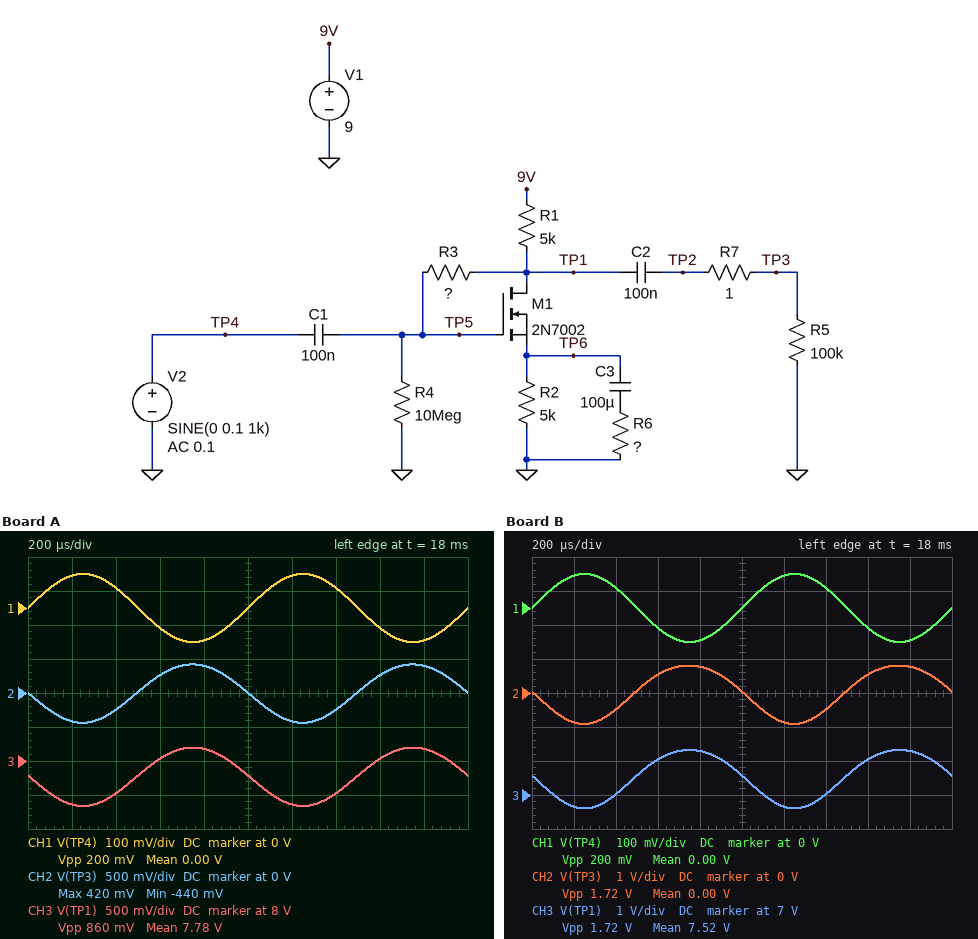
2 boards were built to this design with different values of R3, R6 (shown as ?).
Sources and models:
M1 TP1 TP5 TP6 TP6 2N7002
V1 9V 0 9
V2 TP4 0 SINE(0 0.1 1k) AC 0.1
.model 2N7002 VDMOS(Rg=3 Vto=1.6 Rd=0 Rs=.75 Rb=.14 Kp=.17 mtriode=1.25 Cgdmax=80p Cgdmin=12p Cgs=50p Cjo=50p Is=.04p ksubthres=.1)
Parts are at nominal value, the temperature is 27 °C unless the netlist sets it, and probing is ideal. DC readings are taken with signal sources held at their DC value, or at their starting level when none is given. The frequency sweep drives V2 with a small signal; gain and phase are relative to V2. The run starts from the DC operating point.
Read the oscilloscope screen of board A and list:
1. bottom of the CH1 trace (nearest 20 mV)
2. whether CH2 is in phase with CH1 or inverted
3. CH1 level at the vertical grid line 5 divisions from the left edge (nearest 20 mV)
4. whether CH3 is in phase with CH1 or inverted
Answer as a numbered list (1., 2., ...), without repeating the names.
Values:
1. -100 mV
2. inverted
3. 0 V
4. inverted
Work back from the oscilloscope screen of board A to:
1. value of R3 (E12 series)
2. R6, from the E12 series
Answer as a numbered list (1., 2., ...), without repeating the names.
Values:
1. 18 MΩ
2. 1 kΩ
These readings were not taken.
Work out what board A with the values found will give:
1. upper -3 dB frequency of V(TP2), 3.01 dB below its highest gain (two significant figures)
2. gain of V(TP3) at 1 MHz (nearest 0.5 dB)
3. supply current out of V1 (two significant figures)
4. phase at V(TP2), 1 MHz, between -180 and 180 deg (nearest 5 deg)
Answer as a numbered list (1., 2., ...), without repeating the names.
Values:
1. 1.9 MHz
2. 11.5 dB
3. 240 µA
4. 135 deg
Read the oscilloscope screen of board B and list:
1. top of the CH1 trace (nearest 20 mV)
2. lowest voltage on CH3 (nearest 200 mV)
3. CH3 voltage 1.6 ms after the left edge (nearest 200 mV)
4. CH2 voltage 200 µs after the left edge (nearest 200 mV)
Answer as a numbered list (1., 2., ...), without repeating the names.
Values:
1. 100 mV
2. 6.6 V
3. 8.0 V
4. -800 mV
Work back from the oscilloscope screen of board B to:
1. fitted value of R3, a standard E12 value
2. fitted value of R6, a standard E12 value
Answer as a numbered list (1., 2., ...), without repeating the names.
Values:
1. 15 MΩ
2. 330 Ω
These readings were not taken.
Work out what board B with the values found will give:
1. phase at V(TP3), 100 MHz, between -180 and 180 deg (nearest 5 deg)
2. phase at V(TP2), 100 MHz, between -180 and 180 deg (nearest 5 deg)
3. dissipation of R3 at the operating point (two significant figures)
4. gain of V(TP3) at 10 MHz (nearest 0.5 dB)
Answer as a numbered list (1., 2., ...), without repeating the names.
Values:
1. 5 deg
2. 5 deg
3. 1.4 µW
4. 4.5 dB
